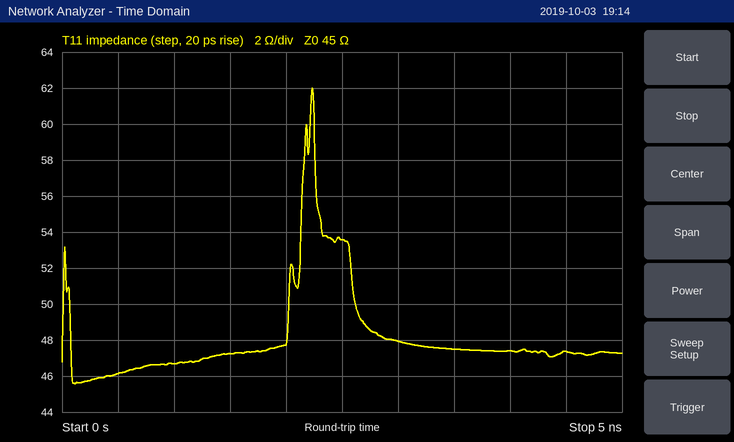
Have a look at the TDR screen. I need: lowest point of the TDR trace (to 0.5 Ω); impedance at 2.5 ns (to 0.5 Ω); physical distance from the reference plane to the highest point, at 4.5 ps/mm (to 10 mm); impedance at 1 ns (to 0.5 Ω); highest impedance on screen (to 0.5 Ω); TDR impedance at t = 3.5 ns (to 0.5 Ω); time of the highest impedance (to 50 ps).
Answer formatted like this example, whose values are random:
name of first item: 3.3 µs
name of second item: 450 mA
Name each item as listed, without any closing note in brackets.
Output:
lowest point of the TDR trace: 45.5 Ω
impedance at 2.5 ns: 53.5 Ω
physical distance from the reference plane to the highest point, at 4.5 ps/mm: 250 mm
impedance at 1 ns: 46.5 Ω
highest impedance on screen: 62.0 Ω
TDR impedance at t = 3.5 ns: 47.5 Ω
time of the highest impedance: 2.25 ns
